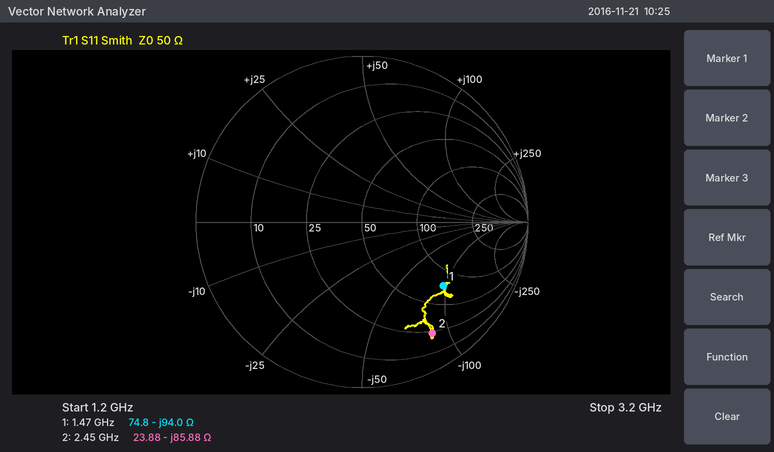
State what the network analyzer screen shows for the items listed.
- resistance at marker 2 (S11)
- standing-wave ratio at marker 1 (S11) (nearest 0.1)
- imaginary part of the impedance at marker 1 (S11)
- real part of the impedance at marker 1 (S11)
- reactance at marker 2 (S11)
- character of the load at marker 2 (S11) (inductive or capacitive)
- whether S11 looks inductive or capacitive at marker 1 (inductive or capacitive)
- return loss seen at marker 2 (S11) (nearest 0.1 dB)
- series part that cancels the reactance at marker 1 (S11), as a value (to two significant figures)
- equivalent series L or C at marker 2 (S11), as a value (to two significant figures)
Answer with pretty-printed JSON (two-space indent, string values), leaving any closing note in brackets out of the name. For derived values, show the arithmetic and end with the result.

{
  "resistance at marker 2": "23.88 Ω",
  "standing-wave ratio at marker 1 (S11)": "4.3",
  "imaginary part of the impedance at marker 1": "-94.0 Ω",
  "real part of the impedance at marker 1": "74.8 Ω",
  "reactance at marker 2": "-85.88 Ω",
  "character of the load at marker 2 (S11)": "capacitive",
  "whether S11 looks inductive or capacitive at marker 1": "capacitive",
  "return loss seen at marker 2 (S11)": "2.0 dB",
  "series part that cancels the reactance at marker 1 (S11), as a value": "L = 94 Ω/(2π × 1.47 GHz) ≈ 10 nH",
  "equivalent series L or C at marker 2 (S11), as a value": "C = 1/(2π × 2.45 GHz × 85.88 Ω) ≈ 756 fF, so 760 fF to two significant figures"
}
